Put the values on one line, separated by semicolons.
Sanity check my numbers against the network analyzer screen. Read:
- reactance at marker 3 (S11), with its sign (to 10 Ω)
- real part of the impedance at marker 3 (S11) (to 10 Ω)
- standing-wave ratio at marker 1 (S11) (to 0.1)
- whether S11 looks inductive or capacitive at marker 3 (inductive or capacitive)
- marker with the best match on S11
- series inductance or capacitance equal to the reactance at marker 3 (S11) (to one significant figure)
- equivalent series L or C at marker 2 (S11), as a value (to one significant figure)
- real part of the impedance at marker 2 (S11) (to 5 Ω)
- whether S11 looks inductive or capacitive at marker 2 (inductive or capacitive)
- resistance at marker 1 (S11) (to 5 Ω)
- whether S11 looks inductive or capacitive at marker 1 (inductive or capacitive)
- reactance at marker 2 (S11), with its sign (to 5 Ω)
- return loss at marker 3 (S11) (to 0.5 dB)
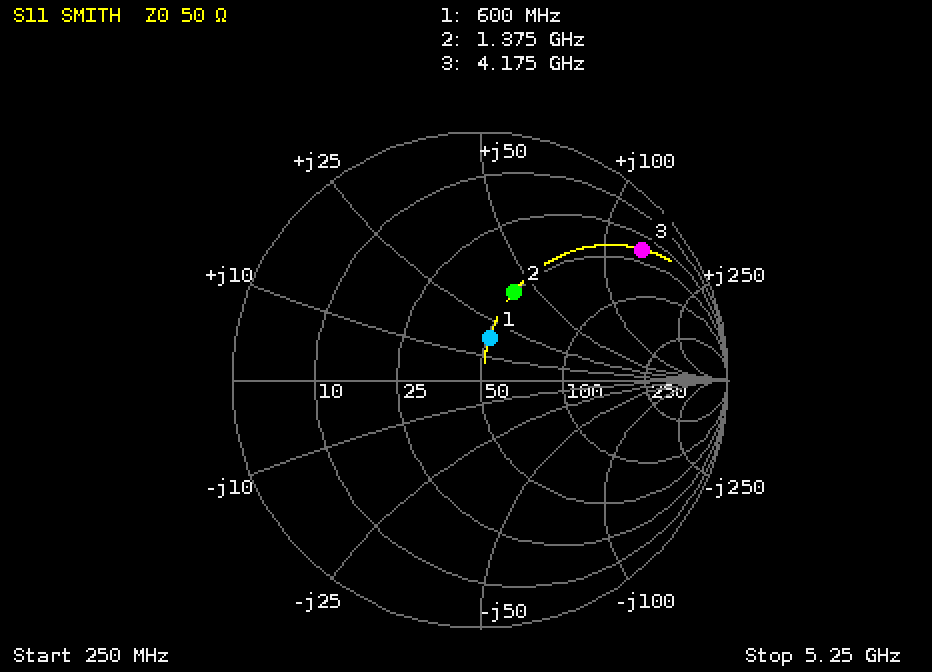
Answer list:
+130 Ω; 40 Ω; 1.4; inductive; marker 1; 5 nH; 5 nH; 50 Ω; inductive; 50 Ω; inductive; +40 Ω; 1.5 dB
